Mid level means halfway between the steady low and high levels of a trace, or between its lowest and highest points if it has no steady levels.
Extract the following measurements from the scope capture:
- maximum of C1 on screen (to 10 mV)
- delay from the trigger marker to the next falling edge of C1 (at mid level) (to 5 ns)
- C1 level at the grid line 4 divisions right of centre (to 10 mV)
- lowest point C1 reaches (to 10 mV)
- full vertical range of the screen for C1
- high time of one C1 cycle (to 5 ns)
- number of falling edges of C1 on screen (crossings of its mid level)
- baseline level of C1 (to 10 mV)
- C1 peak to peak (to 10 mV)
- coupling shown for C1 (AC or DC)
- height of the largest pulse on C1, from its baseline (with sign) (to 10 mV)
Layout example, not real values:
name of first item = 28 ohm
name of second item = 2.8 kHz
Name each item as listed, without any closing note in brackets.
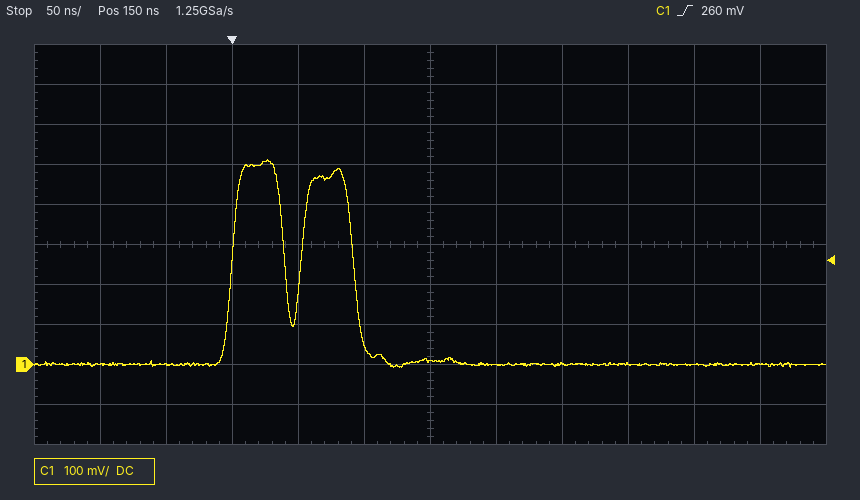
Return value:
maximum of C1 on screen = 510 mV
delay from the trigger marker to the next falling edge of C1 (at mid level) = 40 ns
C1 level at the grid line 4 divisions right of centre = 0 mV
lowest point C1 reaches = -10 mV
full vertical range of the screen for C1 = 1 V
high time of one C1 cycle = 40 ns
number of falling edges of C1 on screen = 2
baseline level of C1 = 0 mV
C1 peak to peak = 520 mV
coupling shown for C1 = DC
height of the largest pulse on C1, from its baseline (with sign) = +510 mV
